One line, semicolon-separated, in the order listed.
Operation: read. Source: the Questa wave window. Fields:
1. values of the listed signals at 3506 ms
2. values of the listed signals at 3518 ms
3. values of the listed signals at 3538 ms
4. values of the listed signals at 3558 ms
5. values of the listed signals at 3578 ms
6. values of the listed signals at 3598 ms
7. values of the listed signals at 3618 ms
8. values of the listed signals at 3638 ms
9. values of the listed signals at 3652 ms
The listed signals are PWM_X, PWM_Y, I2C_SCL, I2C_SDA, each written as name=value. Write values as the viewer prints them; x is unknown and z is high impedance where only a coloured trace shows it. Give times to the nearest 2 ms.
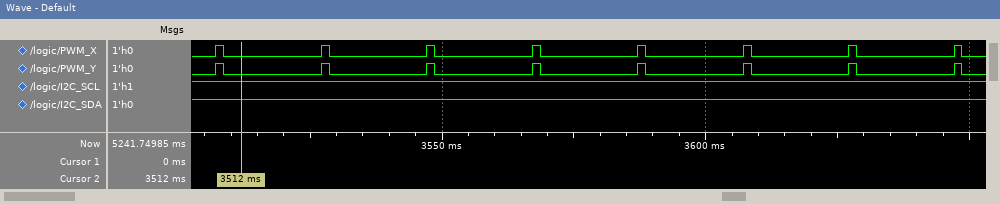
PWM_X=0, PWM_Y=0, I2C_SCL=1, I2C_SDA=1; PWM_X=0, PWM_Y=0, I2C_SCL=1, I2C_SDA=1; PWM_X=0, PWM_Y=0, I2C_SCL=1, I2C_SDA=1; PWM_X=0, PWM_Y=0, I2C_SCL=1, I2C_SDA=1; PWM_X=0, PWM_Y=0, I2C_SCL=1, I2C_SDA=1; PWM_X=0, PWM_Y=0, I2C_SCL=1, I2C_SDA=1; PWM_X=0, PWM_Y=0, I2C_SCL=1, I2C_SDA=1; PWM_X=0, PWM_Y=0, I2C_SCL=1, I2C_SDA=1; PWM_X=0, PWM_Y=0, I2C_SCL=1, I2C_SDA=1
